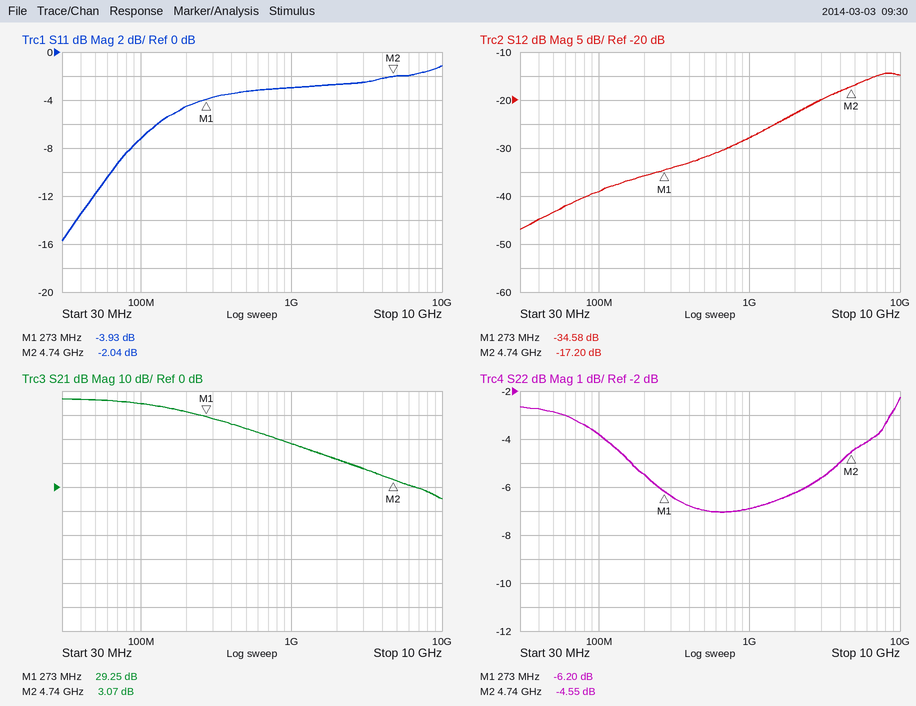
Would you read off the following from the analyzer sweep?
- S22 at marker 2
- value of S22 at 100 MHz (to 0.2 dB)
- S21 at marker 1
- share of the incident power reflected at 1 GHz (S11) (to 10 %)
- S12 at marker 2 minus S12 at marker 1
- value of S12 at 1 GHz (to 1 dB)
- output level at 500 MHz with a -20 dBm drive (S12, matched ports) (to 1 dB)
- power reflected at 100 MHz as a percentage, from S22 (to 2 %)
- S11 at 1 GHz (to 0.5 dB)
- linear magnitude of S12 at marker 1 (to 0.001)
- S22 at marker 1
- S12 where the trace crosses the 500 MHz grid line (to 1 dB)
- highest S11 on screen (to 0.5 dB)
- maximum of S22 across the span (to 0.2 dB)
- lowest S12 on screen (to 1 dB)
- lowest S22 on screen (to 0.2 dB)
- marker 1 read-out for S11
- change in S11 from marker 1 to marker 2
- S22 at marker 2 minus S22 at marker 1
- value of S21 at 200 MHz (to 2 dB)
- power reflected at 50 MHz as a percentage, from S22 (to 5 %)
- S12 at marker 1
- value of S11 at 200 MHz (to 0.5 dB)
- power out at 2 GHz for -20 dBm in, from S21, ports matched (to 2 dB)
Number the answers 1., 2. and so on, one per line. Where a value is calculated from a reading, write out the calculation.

1. -4.55 dB
2. -3.8 dB
3. 29.25 dB
4. 10^(-3/10) ≈ 50 %
5. -17.2 − (-34.58) = 17.38 dB
6. -28 dB
7. -20 dBm + (-32 dB) = -52 dBm
8. 10^(-3.8/10) ≈ 42 %
9. -3.0 dB
10. 10^(-34.58/20) ≈ 0.019
11. -6.20 dB
12. -32 dB
13. -1.0 dB
14. -2.2 dB
15. -47 dB
16. -7.0 dB
17. -3.93 dB
18. -2.04 − (-3.93) = 1.89 dB
19. -4.55 − (-6.2) = 1.65 dB
20. 32 dB
21. 10^(-2.8/10) ≈ 52.5 %, so 50 % to the nearest 5 %
22. -34.58 dB
23. -4.5 dB
24. -20 dBm + (12 dB) = -8 dBm
